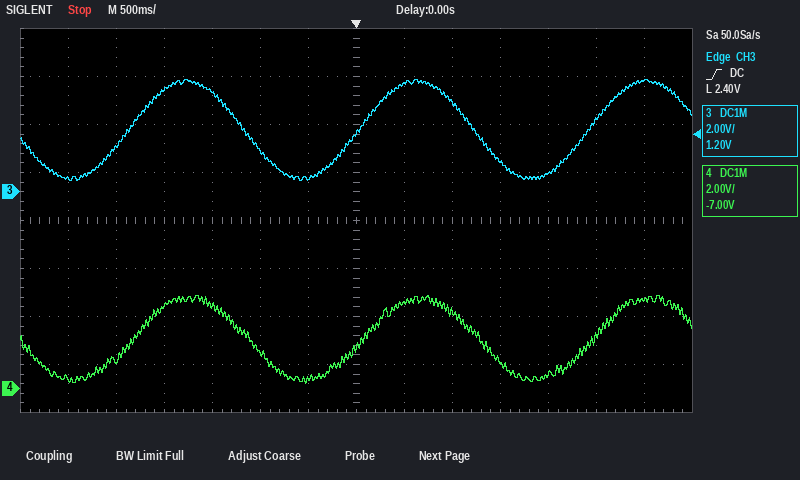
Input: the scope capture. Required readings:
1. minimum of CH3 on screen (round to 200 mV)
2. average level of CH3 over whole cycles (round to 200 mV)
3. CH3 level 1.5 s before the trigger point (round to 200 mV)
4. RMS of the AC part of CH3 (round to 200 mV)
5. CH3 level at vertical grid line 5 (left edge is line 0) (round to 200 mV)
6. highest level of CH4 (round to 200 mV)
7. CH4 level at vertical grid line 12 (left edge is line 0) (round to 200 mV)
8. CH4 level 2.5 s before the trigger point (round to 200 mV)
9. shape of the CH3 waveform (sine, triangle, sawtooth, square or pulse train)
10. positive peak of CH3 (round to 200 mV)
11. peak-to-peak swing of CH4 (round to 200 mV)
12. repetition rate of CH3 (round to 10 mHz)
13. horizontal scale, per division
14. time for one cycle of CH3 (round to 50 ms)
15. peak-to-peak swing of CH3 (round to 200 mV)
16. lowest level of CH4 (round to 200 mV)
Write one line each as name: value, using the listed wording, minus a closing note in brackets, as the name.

minimum of CH3 on screen: 400 mV
average level of CH3 over whole cycles: 2.6 V
CH3 level 1.5 s before the trigger point: 4.2 V
RMS of the AC part of CH3: 1.4 V
CH3 level at vertical grid line 5 (left edge is line 0): 1.6 V
highest level of CH4: 3.8 V
CH4 level at vertical grid line 12 (left edge is line 0): 2.2 V
CH4 level 2.5 s before the trigger point: 1.2 V
shape of the CH3 waveform: sine
positive peak of CH3: 4.6 V
peak-to-peak swing of CH4: 3.6 V
repetition rate of CH3: 420 mHz
horizontal scale, per division: 500 ms
time for one cycle of CH3: 2.40 s
peak-to-peak swing of CH3: 4.2 V
lowest level of CH4: 200 mV
